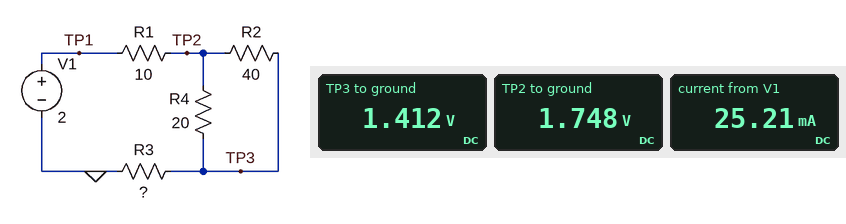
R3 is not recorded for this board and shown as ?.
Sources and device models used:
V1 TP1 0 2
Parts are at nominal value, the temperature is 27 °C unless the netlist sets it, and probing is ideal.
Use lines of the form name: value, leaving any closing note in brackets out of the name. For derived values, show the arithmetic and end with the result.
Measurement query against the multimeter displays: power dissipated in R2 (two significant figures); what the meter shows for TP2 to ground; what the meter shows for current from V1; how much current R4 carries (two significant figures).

power dissipated in R2: (1.748 V - 1.412 V)^2 / 40 Ω = 2.8 mW
what the meter shows for TP2 to ground: 1.748 V
what the meter shows for current from V1: 25.21 mA
how much current R4 carries: (1.748 V - 1.412 V) / 20 Ω = 17 mA
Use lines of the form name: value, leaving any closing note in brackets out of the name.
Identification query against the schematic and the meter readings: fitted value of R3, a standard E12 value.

fitted value of R3, a standard E12 value: 56 Ω
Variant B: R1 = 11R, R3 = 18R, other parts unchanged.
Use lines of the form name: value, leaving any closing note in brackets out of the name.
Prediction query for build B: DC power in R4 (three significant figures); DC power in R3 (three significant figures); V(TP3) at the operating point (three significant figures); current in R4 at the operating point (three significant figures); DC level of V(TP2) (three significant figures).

DC power in R4: 19.8 mW
DC power in R3: 40.2 mW
V(TP3) at the operating point: 850 mV
current in R4 at the operating point: 31.5 mA
DC level of V(TP2): 1.48 V
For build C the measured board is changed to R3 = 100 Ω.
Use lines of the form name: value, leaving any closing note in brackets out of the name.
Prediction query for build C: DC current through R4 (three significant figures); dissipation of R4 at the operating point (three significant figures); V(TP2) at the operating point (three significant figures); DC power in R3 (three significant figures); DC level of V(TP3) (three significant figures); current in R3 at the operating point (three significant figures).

DC current through R4: 10.8 mA
dissipation of R4 at the operating point: 2.34 mW
V(TP2) at the operating point: 1.84 V
DC power in R3: 26.3 mW
DC level of V(TP3): 1.62 V
current in R3 at the operating point: 16.2 mA
